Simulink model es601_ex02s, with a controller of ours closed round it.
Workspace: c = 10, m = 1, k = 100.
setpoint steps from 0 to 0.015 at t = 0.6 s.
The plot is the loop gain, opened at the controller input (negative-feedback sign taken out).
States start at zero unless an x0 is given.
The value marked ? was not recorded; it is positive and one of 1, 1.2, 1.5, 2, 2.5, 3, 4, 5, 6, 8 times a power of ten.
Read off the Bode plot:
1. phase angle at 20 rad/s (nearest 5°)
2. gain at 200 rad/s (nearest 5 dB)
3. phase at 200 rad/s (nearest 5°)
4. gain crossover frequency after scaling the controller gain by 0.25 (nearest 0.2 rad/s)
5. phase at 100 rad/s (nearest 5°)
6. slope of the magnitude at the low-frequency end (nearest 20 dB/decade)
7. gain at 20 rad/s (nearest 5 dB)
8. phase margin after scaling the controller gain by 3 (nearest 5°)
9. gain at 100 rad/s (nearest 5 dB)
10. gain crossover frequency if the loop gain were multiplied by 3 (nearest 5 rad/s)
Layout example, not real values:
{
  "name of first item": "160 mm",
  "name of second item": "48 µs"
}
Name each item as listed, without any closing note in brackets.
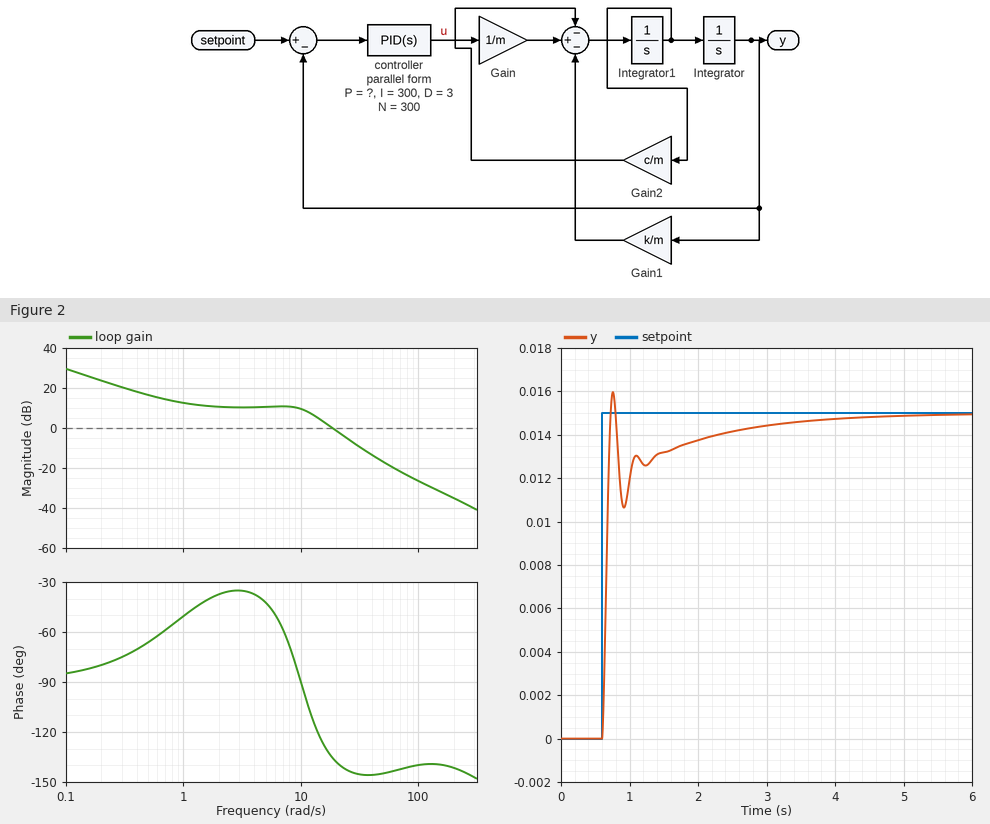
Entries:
{
  "phase angle at 20 rad/s": "-140°",
  "gain at 200 rad/s": "-35 dB",
  "phase at 200 rad/s": "-140°",
  "gain crossover frequency after scaling the controller gain by 0.25": "1.2 rad/s",
  "phase at 100 rad/s": "-140°",
  "slope of the magnitude at the low-frequency end": "-20 dB/decade",
  "gain at 20 rad/s": "0 dB",
  "phase margin after scaling the controller gain by 3": "35°",
  "gain at 100 rad/s": "-25 dB",
  "gain crossover frequency if the loop gain were multiplied by 3": "30 rad/s"
}
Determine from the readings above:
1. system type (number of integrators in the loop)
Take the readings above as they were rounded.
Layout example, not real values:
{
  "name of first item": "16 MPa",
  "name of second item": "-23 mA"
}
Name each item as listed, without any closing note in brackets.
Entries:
{
  "system type": "1"
}
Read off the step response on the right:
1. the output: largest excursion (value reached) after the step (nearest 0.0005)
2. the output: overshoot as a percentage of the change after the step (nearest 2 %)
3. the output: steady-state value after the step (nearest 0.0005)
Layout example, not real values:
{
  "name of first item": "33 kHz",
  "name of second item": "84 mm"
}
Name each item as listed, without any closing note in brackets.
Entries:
{
  "the output: largest excursion (value reached) after the step": "0.0160",
  "the output: overshoot as a percentage of the change after the step": "6 %",
  "the output: steady-state value after the step": "0.0150"
}
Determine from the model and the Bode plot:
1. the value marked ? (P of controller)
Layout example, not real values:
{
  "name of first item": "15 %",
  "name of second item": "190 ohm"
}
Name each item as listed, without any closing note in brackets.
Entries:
{
  "the value marked ?": "300"
}
